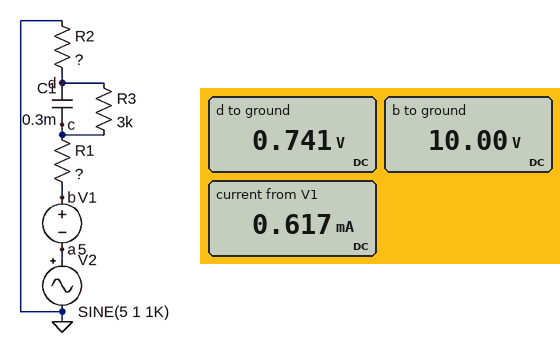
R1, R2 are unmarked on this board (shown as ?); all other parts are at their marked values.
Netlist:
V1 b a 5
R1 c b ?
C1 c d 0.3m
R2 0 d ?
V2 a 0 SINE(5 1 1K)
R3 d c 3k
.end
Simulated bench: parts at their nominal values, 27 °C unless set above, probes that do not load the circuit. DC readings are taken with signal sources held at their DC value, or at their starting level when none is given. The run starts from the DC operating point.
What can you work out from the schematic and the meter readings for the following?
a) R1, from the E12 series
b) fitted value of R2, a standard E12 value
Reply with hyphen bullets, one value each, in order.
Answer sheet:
- 12 kΩ
- 1.2 kΩ
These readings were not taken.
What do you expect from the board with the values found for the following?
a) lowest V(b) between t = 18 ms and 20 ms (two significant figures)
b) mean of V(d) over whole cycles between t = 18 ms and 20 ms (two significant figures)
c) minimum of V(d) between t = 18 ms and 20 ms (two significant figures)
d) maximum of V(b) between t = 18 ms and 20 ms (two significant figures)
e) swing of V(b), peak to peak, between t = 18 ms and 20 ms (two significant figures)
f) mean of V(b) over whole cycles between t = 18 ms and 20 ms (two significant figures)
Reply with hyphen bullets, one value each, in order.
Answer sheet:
- 9.0 V
- 740 mV
- 650 mV
- 11 V
- 2.0 V
- 10 V
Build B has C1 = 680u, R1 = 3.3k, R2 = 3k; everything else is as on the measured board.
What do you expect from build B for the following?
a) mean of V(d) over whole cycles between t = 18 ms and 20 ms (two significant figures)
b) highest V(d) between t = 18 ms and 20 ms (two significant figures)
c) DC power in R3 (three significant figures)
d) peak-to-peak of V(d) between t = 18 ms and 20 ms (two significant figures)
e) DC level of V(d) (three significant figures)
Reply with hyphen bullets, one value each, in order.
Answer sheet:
- 3.2 V
- 3.7 V
- 3.47 mW
- 950 mV
- 3.23 V
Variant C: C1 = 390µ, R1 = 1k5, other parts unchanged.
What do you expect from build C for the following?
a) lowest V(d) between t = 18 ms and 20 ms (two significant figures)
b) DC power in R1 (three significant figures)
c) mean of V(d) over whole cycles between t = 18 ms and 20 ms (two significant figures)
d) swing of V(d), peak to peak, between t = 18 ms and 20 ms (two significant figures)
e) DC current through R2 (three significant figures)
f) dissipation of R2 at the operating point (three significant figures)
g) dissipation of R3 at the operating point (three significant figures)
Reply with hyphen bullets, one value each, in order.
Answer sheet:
- 1.7 V
- 4.62 mW
- 2.1 V
- 890 mV
- 1.75 mA
- 3.69 mW
- 9.23 mW
